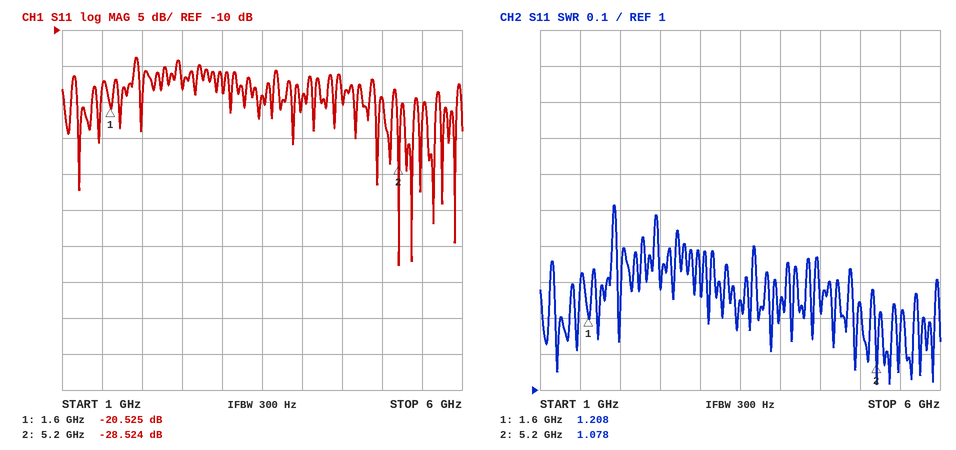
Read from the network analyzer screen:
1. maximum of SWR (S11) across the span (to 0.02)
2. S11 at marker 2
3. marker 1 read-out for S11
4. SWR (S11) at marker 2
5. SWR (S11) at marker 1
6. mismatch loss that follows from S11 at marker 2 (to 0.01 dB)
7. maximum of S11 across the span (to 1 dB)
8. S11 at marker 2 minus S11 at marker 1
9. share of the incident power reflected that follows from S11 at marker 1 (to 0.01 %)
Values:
1.52
-28.524 dB
-20.525 dB
1.078
1.208
0.01 dB
-14 dB
-7.999 dB
0.89 %
